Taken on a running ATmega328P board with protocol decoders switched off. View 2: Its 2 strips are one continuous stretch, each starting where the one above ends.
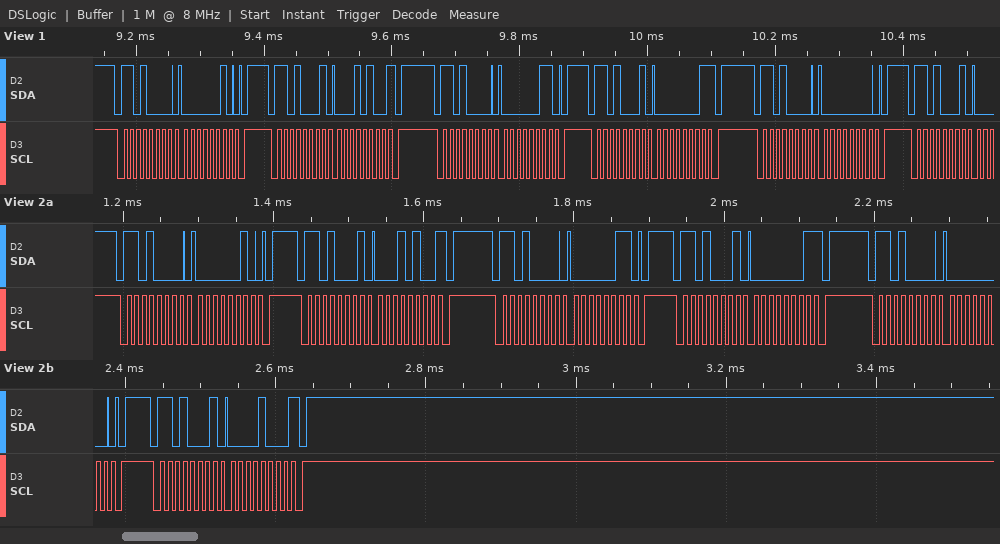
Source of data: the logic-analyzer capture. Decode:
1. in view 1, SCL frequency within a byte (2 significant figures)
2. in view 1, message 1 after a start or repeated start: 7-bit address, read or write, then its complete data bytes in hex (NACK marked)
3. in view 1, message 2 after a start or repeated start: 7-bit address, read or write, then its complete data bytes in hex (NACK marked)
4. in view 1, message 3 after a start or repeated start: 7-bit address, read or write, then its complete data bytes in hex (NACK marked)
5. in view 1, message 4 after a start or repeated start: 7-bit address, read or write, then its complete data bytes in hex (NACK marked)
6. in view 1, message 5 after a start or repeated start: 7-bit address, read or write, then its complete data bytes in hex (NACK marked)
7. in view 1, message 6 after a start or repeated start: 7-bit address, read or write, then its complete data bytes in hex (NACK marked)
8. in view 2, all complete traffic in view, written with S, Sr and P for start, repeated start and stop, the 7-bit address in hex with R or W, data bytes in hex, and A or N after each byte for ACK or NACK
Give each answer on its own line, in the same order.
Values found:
100 kHz
0x68 write: 02
0x68 read: 14 NACK
0x68 write: 03
0x68 read: 01 NACK
0x68 write: 00
0x68 read
S 68W A 02 A P S 68R A 14 N P S 68W A 03 A P S 68R A 01 N P S 68W A 00 A P S 68R A 08 N P
